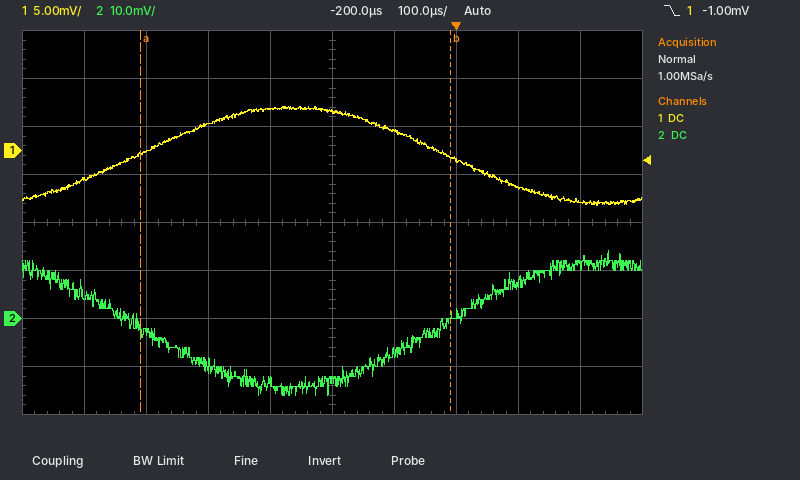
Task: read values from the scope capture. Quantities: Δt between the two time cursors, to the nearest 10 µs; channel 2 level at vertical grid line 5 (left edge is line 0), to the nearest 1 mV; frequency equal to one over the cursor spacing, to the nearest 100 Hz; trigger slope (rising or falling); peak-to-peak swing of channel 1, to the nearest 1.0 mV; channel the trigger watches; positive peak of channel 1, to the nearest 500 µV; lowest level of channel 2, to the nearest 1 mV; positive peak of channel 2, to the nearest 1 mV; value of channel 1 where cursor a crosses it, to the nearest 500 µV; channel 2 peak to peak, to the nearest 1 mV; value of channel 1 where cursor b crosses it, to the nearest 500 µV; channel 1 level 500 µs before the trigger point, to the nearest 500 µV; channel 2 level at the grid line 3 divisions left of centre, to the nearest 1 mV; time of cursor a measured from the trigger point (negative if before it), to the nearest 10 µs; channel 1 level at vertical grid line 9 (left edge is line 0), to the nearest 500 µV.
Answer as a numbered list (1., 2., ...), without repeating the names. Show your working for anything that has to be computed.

1. 500 µs
2. -13 mV
3. 1 / 500 µs ≈ 2.0 kHz
4. falling
5. 10.0 mV
6. channel 1
7. 4.5 mV
8. -16 mV
9. 14 mV
10. -500 µV
11. 14 mV − (-16 mV) = 30 mV
12. -500 µV
13. 0.0 mV
14. -3 mV
15. -510 µs
16. -5.5 mV
